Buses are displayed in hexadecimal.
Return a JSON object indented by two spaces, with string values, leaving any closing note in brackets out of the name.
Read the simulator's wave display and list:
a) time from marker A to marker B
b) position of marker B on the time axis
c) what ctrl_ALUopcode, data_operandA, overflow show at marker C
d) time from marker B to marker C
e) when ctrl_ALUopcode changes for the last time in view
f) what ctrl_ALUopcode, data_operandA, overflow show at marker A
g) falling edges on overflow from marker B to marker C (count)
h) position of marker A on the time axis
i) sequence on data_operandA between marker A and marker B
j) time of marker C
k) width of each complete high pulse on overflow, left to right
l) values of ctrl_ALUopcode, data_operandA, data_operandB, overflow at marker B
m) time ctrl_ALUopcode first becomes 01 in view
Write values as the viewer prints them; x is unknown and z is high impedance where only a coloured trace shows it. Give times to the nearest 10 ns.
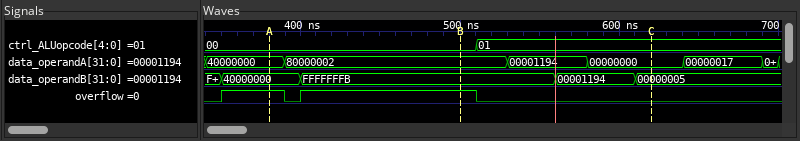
{
  "time from marker A to marker B": "120 ns",
  "position of marker B on the time axis": "500 ns",
  "what ctrl_ALUopcode, data_operandA, overflow show at marker C": "ctrl_ALUopcode=01, data_operandA=00000000, overflow=0",
  "time from marker B to marker C": "120 ns",
  "when ctrl_ALUopcode changes for the last time in view": "510 ns",
  "what ctrl_ALUopcode, data_operandA, overflow show at marker A": "ctrl_ALUopcode=00, data_operandA=40000000, overflow=1",
  "falling edges on overflow from marker B to marker C": "1",
  "position of marker A on the time axis": "380 ns",
  "sequence on data_operandA between marker A and marker B": "40000000, 80000002",
  "time of marker C": "620 ns",
  "width of each complete high pulse on overflow, left to right": "40 ns, 110 ns",
  "values of ctrl_ALUopcode, data_operandA, data_operandB, overflow at marker B": "ctrl_ALUopcode=00, data_operandA=80000002, data_operandB=FFFFFFFB, overflow=1",
  "time ctrl_ALUopcode first becomes 01 in view": "510 ns"
}
